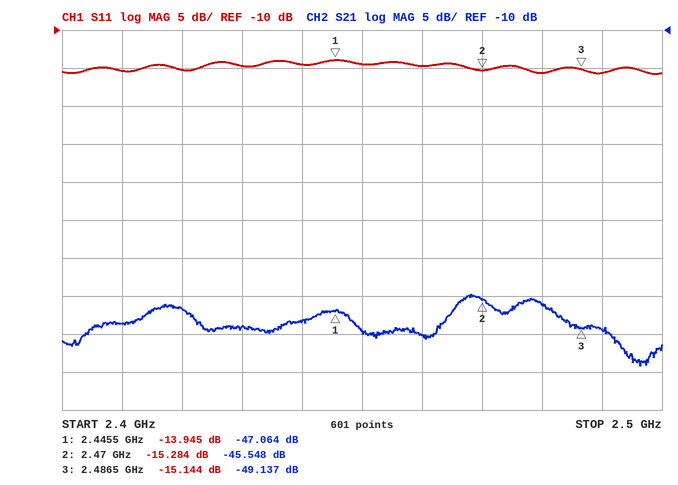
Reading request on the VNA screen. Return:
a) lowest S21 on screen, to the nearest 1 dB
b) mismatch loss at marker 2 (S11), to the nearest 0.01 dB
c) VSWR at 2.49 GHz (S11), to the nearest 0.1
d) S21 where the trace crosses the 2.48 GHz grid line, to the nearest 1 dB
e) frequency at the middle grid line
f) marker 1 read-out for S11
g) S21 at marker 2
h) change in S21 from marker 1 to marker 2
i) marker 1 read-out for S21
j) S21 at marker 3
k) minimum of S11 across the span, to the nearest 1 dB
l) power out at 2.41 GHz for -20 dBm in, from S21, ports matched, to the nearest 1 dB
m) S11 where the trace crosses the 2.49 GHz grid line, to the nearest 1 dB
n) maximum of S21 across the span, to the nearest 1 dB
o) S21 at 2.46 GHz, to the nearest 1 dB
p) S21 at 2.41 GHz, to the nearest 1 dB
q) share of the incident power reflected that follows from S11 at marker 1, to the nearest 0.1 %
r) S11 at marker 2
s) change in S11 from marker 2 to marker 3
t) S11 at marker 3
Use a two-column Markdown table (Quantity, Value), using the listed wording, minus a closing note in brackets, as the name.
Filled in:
| Quantity | Value |
|---|---|
| lowest S21 on screen, to the nearest 1 dB | -54 dB |
| mismatch loss at marker 2 (S11), to the nearest 0.01 dB | 0.13 dB |
| VSWR at 2.49 GHz (S11), to the nearest 0.1 | 1.4 |
| S21 where the trace crosses the 2.48 GHz grid line, to the nearest 1 dB | -46 dB |
| frequency at the middle grid line | 2.45 GHz |
| marker 1 read-out for S11 | -13.945 dB |
| S21 at marker 2 | -45.548 dB |
| change in S21 from marker 1 to marker 2 | 1.516 dB |
| marker 1 read-out for S21 | -47.064 dB |
| S21 at marker 3 | -49.137 dB |
| minimum of S11 across the span, to the nearest 1 dB | -16 dB |
| power out at 2.41 GHz for -20 dBm in, from S21, ports matched, to the nearest 1 dB | -69 dBm |
| S11 where the trace crosses the 2.49 GHz grid line, to the nearest 1 dB | -16 dB |
| maximum of S21 across the span, to the nearest 1 dB | -45 dB |
| S21 at 2.46 GHz, to the nearest 1 dB | -50 dB |
| S21 at 2.41 GHz, to the nearest 1 dB | -49 dB |
| share of the incident power reflected that follows from S11 at marker 1, to the nearest 0.1 % | 4.0 % |
| S11 at marker 2 | -15.284 dB |
| change in S11 from marker 2 to marker 3 | 0.140 dB |
| S11 at marker 3 | -15.144 dB |
